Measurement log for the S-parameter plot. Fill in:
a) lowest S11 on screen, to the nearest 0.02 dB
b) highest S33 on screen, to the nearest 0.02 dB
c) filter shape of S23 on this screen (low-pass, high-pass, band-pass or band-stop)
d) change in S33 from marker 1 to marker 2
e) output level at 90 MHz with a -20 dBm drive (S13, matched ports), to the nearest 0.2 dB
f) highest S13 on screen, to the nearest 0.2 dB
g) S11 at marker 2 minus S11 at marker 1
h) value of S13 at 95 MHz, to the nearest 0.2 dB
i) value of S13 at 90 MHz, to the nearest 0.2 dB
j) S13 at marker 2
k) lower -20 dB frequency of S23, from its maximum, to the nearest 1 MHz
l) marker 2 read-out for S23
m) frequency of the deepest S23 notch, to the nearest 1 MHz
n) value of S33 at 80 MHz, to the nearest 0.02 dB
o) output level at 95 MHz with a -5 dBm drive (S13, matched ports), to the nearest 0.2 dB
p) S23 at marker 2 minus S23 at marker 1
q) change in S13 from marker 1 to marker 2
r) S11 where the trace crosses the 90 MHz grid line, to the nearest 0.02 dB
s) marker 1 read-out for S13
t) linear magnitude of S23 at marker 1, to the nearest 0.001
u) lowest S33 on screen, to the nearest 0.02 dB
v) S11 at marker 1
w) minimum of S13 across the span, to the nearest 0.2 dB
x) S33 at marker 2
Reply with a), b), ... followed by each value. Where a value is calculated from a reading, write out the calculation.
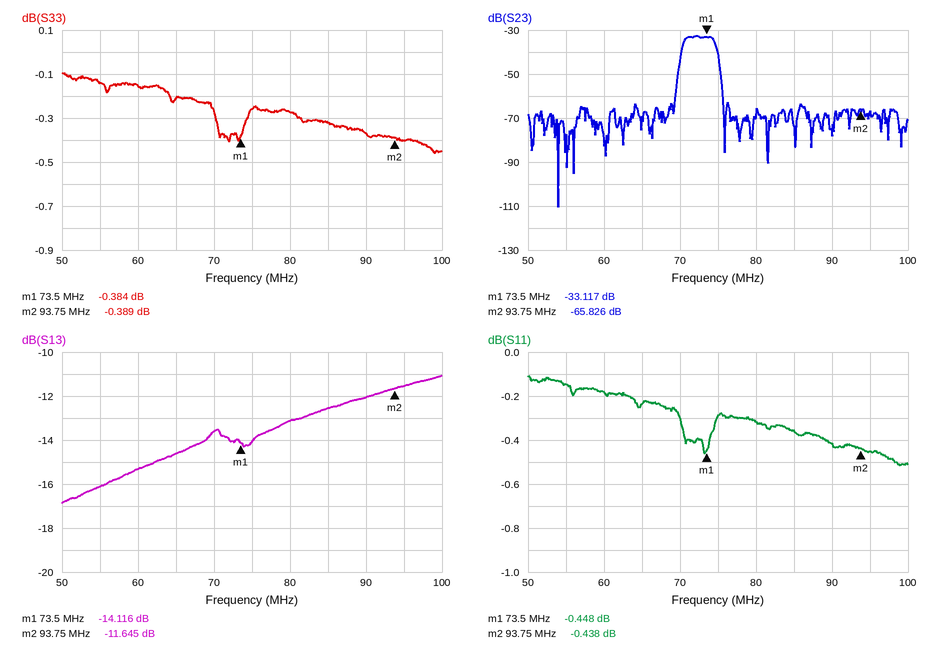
a) -0.52 dB
b) -0.10 dB
c) band-pass
d) -0.389 − (-0.384) = -0.005 dB
e) -20 dBm + (-12.0 dB) = -32.0 dBm
f) -11.0 dB
g) -0.438 − (-0.448) = 0.010 dB
h) -11.6 dB
i) -12.0 dB
j) -11.645 dB
k) 70 MHz
l) -65.826 dB
m) 54 MHz
n) -0.28 dB
o) -5 dBm + (-11.6 dB) = -16.6 dBm
p) -65.826 − (-33.117) = -32.709 dB
q) -11.645 − (-14.116) = 2.471 dB
r) -0.42 dB
s) -14.116 dB
t) 10^(-33.117/20) ≈ 0.022
u) -0.46 dB
v) -0.448 dB
w) -16.8 dB
x) -0.389 dB
